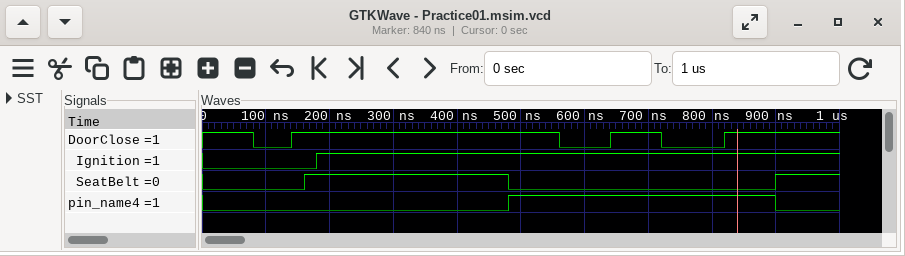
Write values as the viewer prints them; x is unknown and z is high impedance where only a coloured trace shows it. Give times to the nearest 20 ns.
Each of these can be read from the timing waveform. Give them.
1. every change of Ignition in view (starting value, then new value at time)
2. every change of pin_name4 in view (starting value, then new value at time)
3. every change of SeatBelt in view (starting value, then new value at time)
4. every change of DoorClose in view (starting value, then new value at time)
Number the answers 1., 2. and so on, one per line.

1. 0, 1 at 180 ns
2. 0, 1 at 480 ns, 0 at 900 ns
3. 0, 1 at 160 ns, 0 at 480 ns, 1 at 900 ns
4. 1, 0 at 80 ns, 1 at 140 ns, 0 at 560 ns, 1 at 640 ns, 0 at 720 ns, 1 at 820 ns
